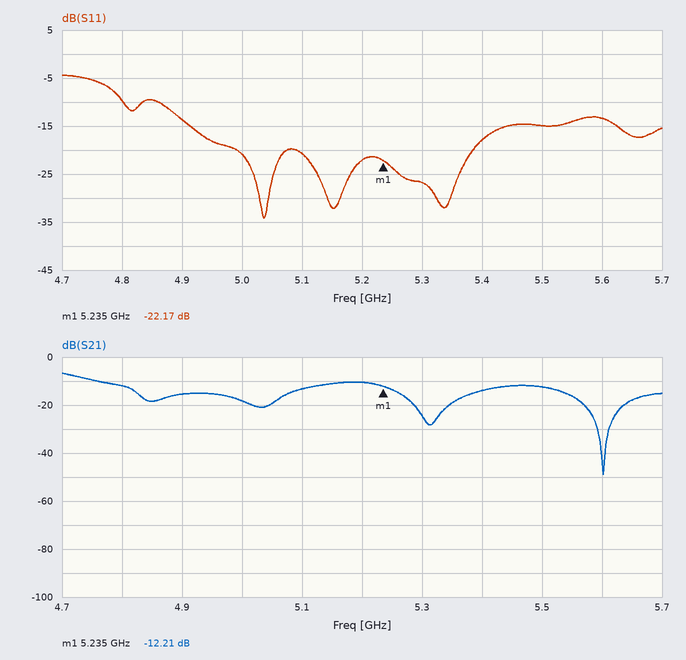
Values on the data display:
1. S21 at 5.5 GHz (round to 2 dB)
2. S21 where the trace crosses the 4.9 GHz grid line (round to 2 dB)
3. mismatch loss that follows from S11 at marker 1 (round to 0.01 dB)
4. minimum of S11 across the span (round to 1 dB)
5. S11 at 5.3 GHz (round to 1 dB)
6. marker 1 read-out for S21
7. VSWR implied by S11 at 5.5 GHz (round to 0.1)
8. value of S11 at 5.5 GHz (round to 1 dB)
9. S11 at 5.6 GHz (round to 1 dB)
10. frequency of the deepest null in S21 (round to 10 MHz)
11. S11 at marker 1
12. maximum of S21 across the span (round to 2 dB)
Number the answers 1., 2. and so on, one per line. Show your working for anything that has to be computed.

1. -12 dB
2. -16 dB
3. −10 log10(1 − 10^(-22.17/10)) ≈ 0.03 dB
4. -34 dB
5. -27 dB
6. -12.21 dB
7. |Γ| = 10^(-15/20) = 0.1778; VSWR = (1 + 0.1778)/(1 − 0.1778) ≈ 1.4
8. -15 dB
9. -13 dB
10. 5.60 GHz
11. -22.17 dB
12. -6 dB
